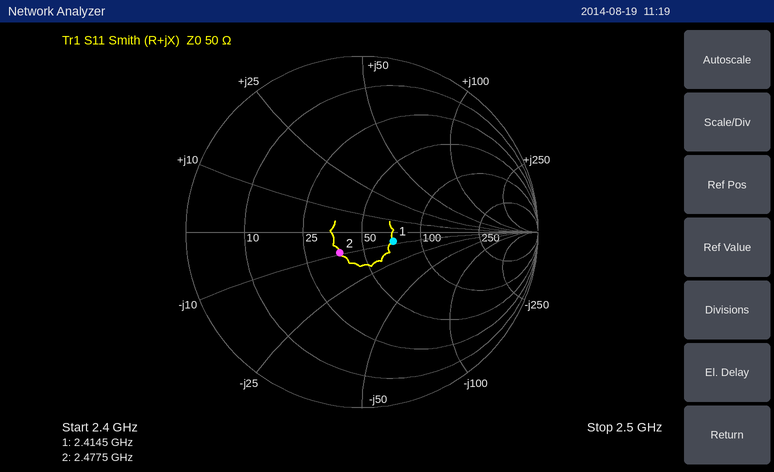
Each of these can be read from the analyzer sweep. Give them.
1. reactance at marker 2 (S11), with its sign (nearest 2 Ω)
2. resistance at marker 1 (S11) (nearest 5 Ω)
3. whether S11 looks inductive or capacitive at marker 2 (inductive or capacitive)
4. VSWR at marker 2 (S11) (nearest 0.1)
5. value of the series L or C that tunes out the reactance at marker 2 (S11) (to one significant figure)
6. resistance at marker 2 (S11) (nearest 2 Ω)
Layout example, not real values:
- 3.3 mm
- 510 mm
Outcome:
- -10 Ω
- 70 Ω
- capacitive
- 1.4
- 600 pH
- 38 Ω
